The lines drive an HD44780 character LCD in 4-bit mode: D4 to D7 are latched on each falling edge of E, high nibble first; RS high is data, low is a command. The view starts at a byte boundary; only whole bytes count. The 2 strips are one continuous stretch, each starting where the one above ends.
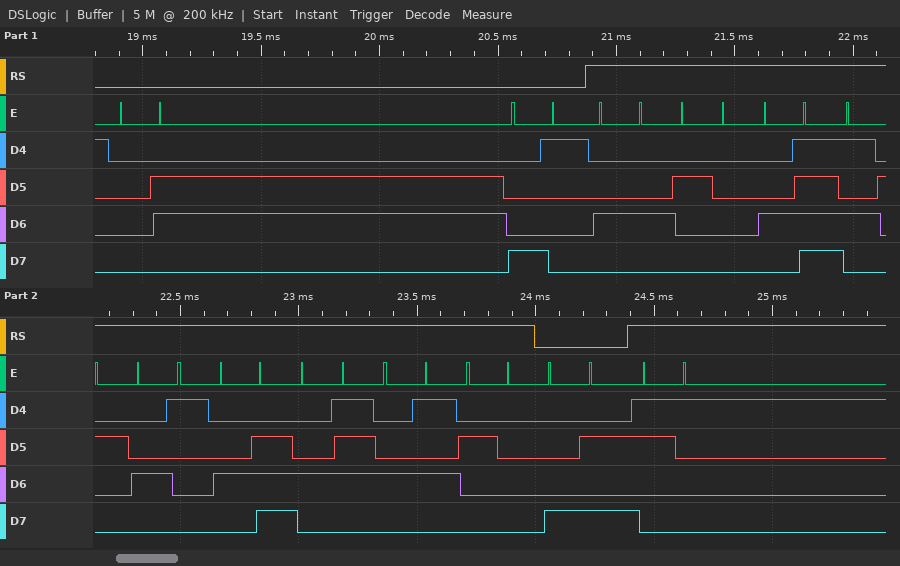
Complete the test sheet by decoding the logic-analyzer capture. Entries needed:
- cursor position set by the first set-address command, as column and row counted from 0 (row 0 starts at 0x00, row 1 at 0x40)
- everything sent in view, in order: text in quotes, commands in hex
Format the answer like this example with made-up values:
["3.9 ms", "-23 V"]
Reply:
["column 1, row 0", "0x06 0x81 \"D ORANGE \" 0x8A \"1\""]
